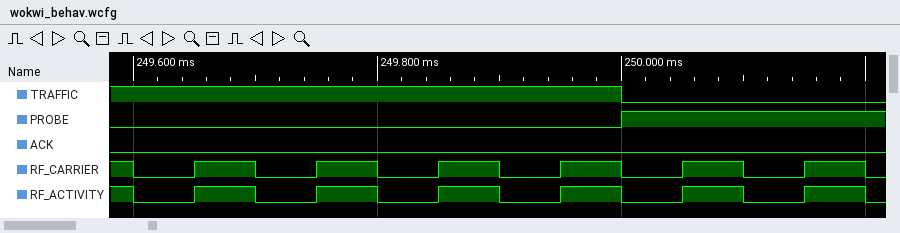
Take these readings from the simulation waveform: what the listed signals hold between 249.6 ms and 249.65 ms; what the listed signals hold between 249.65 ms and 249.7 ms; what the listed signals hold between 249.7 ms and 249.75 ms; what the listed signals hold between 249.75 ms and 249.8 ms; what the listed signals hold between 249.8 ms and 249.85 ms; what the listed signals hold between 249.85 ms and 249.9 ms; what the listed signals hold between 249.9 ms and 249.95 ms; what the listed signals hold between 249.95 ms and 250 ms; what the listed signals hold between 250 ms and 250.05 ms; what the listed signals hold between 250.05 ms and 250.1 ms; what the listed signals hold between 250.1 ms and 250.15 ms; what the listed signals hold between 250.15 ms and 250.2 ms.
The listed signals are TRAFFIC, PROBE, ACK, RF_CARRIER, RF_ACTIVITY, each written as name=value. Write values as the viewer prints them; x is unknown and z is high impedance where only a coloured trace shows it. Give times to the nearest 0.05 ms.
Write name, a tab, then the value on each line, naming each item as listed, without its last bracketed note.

what the listed signals hold between 249.6 ms and 249.65 ms	TRAFFIC=1, PROBE=0, ACK=0, RF_CARRIER=0, RF_ACTIVITY=0
what the listed signals hold between 249.65 ms and 249.7 ms	TRAFFIC=1, PROBE=0, ACK=0, RF_CARRIER=1, RF_ACTIVITY=1
what the listed signals hold between 249.7 ms and 249.75 ms	TRAFFIC=1, PROBE=0, ACK=0, RF_CARRIER=0, RF_ACTIVITY=0
what the listed signals hold between 249.75 ms and 249.8 ms	TRAFFIC=1, PROBE=0, ACK=0, RF_CARRIER=1, RF_ACTIVITY=1
what the listed signals hold between 249.8 ms and 249.85 ms	TRAFFIC=1, PROBE=0, ACK=0, RF_CARRIER=0, RF_ACTIVITY=0
what the listed signals hold between 249.85 ms and 249.9 ms	TRAFFIC=1, PROBE=0, ACK=0, RF_CARRIER=1, RF_ACTIVITY=1
what the listed signals hold between 249.9 ms and 249.95 ms	TRAFFIC=1, PROBE=0, ACK=0, RF_CARRIER=0, RF_ACTIVITY=0
what the listed signals hold between 249.95 ms and 250 ms	TRAFFIC=1, PROBE=0, ACK=0, RF_CARRIER=1, RF_ACTIVITY=1
what the listed signals hold between 250 ms and 250.05 ms	TRAFFIC=0, PROBE=1, ACK=0, RF_CARRIER=0, RF_ACTIVITY=0
what the listed signals hold between 250.05 ms and 250.1 ms	TRAFFIC=0, PROBE=1, ACK=0, RF_CARRIER=1, RF_ACTIVITY=1
what the listed signals hold between 250.1 ms and 250.15 ms	TRAFFIC=0, PROBE=1, ACK=0, RF_CARRIER=0, RF_ACTIVITY=0
what the listed signals hold between 250.15 ms and 250.2 ms	TRAFFIC=0, PROBE=1, ACK=0, RF_CARRIER=1, RF_ACTIVITY=1
